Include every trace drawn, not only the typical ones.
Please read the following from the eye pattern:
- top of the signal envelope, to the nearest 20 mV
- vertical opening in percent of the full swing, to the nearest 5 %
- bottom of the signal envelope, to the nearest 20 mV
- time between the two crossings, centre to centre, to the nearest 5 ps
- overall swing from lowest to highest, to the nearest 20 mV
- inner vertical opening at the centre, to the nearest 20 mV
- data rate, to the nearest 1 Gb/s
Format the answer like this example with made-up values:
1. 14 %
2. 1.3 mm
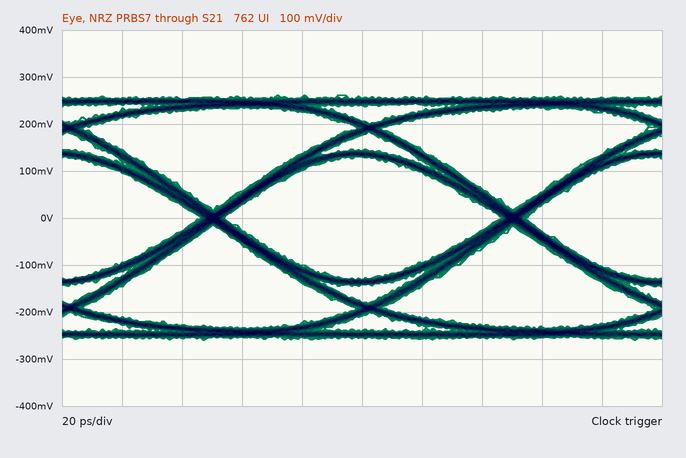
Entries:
1. 260 mV
2. 50 %
3. -260 mV
4. 100 ps
5. 520 mV
6. 260 mV
7. 10 Gb/s
